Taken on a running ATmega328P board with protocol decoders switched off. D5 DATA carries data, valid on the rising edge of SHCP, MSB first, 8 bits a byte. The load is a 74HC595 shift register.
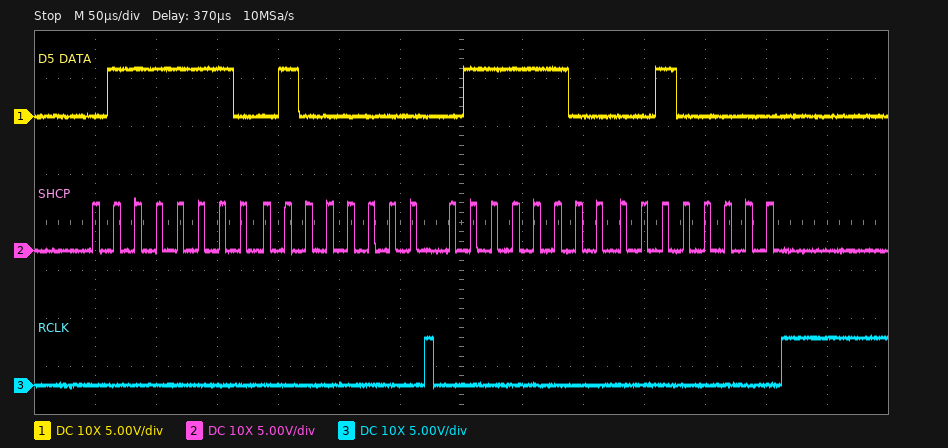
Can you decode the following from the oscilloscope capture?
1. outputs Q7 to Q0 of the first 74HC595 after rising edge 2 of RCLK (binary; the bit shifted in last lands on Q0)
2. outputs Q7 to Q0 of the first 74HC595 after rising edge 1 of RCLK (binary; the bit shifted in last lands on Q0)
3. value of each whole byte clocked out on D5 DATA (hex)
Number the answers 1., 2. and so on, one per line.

1. 00100000
2. 01000000
3. 7E 40 7C 20
